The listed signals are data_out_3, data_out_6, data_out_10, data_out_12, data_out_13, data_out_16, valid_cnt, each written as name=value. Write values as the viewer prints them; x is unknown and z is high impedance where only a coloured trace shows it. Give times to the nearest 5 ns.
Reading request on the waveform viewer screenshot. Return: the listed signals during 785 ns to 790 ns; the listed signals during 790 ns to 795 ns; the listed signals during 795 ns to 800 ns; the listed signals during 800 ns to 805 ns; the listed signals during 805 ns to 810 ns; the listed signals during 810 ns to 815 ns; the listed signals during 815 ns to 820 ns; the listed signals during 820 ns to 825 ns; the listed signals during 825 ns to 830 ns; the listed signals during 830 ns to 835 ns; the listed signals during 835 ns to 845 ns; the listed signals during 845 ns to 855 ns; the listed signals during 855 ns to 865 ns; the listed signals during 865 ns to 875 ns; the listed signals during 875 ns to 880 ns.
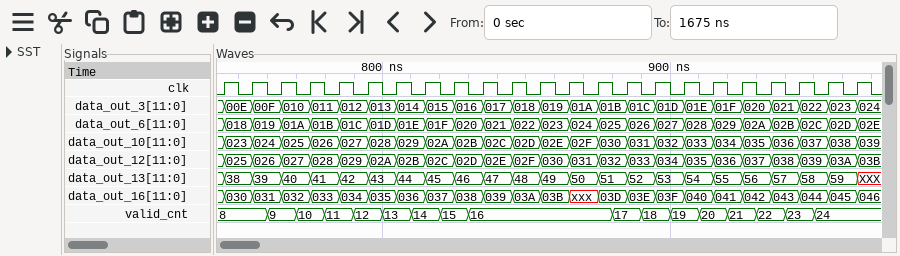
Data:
data_out_3=012, data_out_6=01C, data_out_10=027, data_out_12=029, data_out_13=42, data_out_16=034, valid_cnt=11
data_out_3=012, data_out_6=01C, data_out_10=027, data_out_12=029, data_out_13=42, data_out_16=034, valid_cnt=12
data_out_3=013, data_out_6=01D, data_out_10=028, data_out_12=02A, data_out_13=43, data_out_16=035, valid_cnt=12
data_out_3=013, data_out_6=01D, data_out_10=028, data_out_12=02A, data_out_13=43, data_out_16=035, valid_cnt=13
data_out_3=014, data_out_6=01E, data_out_10=029, data_out_12=02B, data_out_13=44, data_out_16=036, valid_cnt=13
data_out_3=014, data_out_6=01E, data_out_10=029, data_out_12=02B, data_out_13=44, data_out_16=036, valid_cnt=14
data_out_3=015, data_out_6=01F, data_out_10=02A, data_out_12=02C, data_out_13=45, data_out_16=037, valid_cnt=14
data_out_3=015, data_out_6=01F, data_out_10=02A, data_out_12=02C, data_out_13=45, data_out_16=037, valid_cnt=15
data_out_3=016, data_out_6=020, data_out_10=02B, data_out_12=02D, data_out_13=46, data_out_16=038, valid_cnt=15
data_out_3=016, data_out_6=020, data_out_10=02B, data_out_12=02D, data_out_13=46, data_out_16=038, valid_cnt=16
data_out_3=017, data_out_6=021, data_out_10=02C, data_out_12=02E, data_out_13=47, data_out_16=039, valid_cnt=16
data_out_3=018, data_out_6=022, data_out_10=02D, data_out_12=02F, data_out_13=48, data_out_16=03A, valid_cnt=16
data_out_3=019, data_out_6=023, data_out_10=02E, data_out_12=030, data_out_13=49, data_out_16=03B, valid_cnt=16
data_out_3=01A, data_out_6=024, data_out_10=02F, data_out_12=031, data_out_13=50, data_out_16=xxx, valid_cnt=16
data_out_3=01B, data_out_6=025, data_out_10=030, data_out_12=032, data_out_13=51, data_out_16=03D, valid_cnt=16
